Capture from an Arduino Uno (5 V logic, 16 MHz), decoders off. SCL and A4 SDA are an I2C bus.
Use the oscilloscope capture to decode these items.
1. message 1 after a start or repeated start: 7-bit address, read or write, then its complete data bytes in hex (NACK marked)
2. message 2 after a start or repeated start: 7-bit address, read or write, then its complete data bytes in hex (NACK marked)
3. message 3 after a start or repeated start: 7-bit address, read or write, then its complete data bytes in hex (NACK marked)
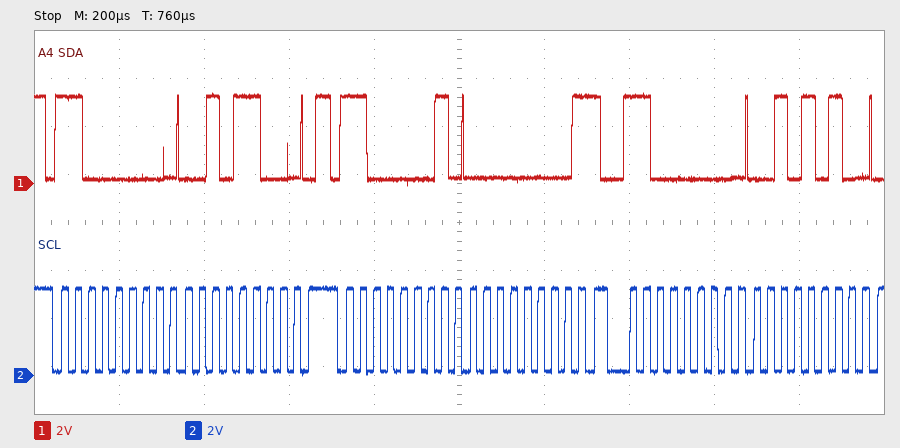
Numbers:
0x60 write: 2C
0x60 read: 00 NACK
0x60 write: 2A
